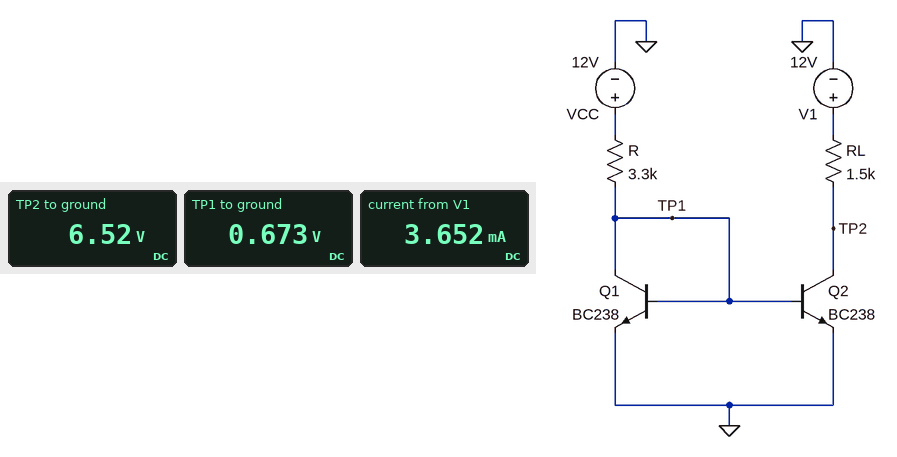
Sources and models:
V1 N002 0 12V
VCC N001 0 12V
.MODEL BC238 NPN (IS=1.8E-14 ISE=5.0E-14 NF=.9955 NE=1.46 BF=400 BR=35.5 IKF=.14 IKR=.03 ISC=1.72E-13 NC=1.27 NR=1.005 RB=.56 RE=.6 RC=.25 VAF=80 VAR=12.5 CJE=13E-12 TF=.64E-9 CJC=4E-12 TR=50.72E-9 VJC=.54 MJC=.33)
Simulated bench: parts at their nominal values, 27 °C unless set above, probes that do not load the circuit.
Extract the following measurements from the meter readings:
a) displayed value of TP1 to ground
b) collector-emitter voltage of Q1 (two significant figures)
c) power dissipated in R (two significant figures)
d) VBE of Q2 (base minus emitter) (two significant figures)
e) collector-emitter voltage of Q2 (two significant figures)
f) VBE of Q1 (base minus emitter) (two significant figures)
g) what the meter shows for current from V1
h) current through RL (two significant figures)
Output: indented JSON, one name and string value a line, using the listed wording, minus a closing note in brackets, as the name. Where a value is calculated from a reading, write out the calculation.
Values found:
{
  "displayed value of TP1 to ground": "0.673 V",
  "collector-emitter voltage of Q1": "673 mV = 670 mV",
  "power dissipated in R": "(12 V - 673 mV)^2 / 3.3 kΩ = 39 mW",
  "VBE of Q2 (base minus emitter)": "673 mV = 670 mV",
  "collector-emitter voltage of Q2": "6.52 V = 6.5 V",
  "VBE of Q1 (base minus emitter)": "673 mV = 670 mV",
  "what the meter shows for current from V1": "3.652 mA",
  "current through RL": "(12 V - 6.52 V) / 1.5 kΩ = 3.7 mA"
}
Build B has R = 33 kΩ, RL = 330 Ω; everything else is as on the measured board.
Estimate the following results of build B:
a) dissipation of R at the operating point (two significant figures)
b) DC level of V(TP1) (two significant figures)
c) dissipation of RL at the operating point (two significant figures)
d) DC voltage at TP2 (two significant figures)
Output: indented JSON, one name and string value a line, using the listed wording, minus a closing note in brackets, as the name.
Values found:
{
  "dissipation of R at the operating point": "3.9 mW",
  "DC level of V(TP1)": "610 mV",
  "dissipation of RL at the operating point": "51 µW",
  "DC voltage at TP2": "12 V"
}
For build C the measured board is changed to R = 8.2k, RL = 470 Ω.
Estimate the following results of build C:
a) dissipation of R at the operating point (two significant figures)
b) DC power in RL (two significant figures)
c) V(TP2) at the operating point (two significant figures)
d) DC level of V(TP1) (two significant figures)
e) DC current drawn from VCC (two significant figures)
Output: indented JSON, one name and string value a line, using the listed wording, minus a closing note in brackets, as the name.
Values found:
{
  "dissipation of R at the operating point": "16 mW",
  "DC power in RL": "1.1 mW",
  "V(TP2) at the operating point": "11 V",
  "DC level of V(TP1)": "650 mV",
  "DC current drawn from VCC": "1.4 mA"
}
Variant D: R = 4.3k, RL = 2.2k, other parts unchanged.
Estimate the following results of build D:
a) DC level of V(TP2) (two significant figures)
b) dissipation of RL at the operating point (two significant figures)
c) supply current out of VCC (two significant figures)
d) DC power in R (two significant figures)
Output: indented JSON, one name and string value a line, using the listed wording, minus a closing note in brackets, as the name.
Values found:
{
  "DC level of V(TP2)": "5.9 V",
  "dissipation of RL at the operating point": "17 mW",
  "supply current out of VCC": "2.6 mA",
  "DC power in R": "30 mW"
}
